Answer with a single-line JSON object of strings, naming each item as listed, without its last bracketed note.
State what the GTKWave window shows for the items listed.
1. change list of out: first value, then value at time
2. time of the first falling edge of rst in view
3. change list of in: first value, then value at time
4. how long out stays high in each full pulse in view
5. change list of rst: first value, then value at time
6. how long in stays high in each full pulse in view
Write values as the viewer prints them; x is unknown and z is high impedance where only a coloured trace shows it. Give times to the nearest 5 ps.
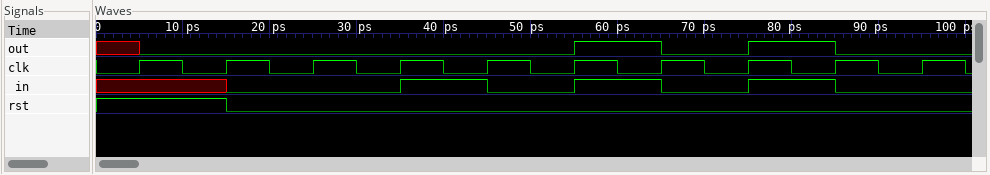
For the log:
{"change list of out: first value, then value at time": "x, 0 at 5 ps, 1 at 55 ps, 0 at 65 ps, 1 at 75 ps, 0 at 85 ps", "time of the first falling edge of rst in view": "15 ps", "change list of in: first value, then value at time": "x, 0 at 15 ps, 1 at 35 ps, 0 at 45 ps, 1 at 55 ps, 0 at 65 ps, 1 at 75 ps, 0 at 85 ps", "how long out stays high in each full pulse in view": "10 ps, 10 ps", "change list of rst: first value, then value at time": "1, 0 at 15 ps", "how long in stays high in each full pulse in view": "10 ps, 10 ps, 10 ps"}
